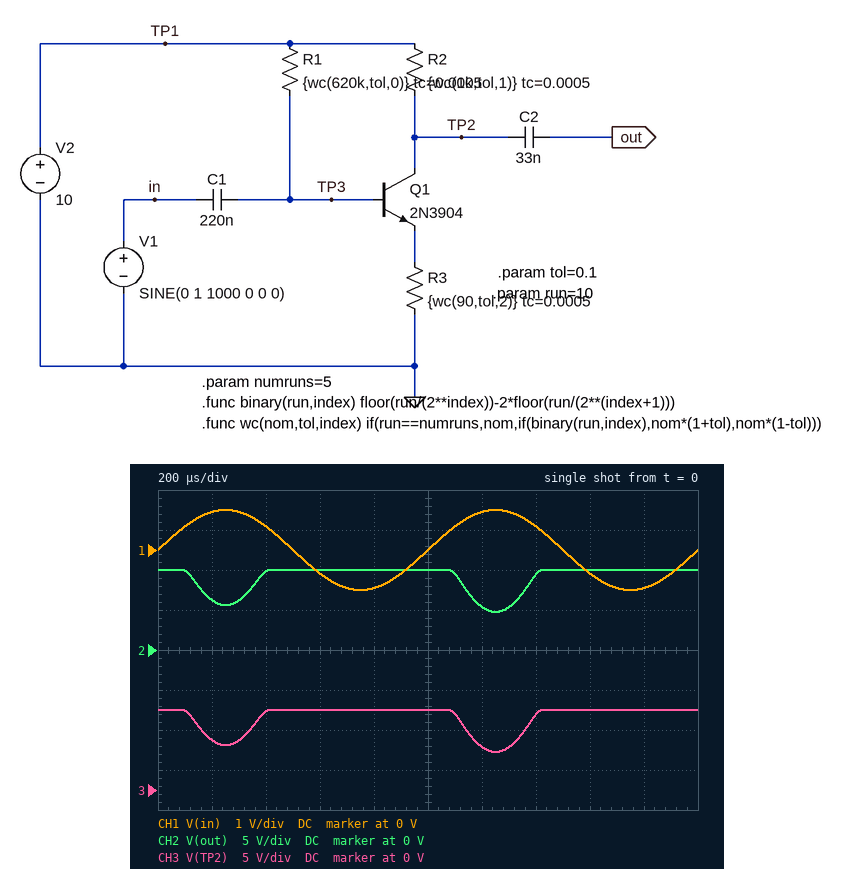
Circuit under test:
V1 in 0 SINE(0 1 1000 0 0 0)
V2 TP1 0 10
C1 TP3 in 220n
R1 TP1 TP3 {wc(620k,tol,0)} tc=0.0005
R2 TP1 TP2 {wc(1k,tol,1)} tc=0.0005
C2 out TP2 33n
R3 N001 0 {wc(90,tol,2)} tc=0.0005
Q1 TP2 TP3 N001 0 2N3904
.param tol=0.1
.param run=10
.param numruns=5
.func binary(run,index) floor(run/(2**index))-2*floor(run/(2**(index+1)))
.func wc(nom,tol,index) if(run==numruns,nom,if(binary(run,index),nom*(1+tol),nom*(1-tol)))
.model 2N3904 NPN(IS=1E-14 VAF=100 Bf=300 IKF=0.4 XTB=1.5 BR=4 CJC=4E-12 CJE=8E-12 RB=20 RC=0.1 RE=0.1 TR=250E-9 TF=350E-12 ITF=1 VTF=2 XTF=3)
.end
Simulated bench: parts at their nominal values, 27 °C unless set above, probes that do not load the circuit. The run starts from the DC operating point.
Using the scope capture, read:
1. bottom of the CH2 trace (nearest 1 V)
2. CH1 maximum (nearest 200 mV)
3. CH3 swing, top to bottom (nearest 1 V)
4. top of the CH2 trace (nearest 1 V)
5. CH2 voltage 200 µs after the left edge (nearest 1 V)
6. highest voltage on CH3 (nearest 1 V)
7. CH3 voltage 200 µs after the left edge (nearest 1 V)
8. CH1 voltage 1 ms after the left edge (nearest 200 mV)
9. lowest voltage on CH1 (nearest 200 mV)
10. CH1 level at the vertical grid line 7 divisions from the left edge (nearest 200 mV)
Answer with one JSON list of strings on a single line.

["5 V", "1.0 V", "5 V", "10 V", "6 V", "10 V", "6 V", "0 V", "-1.0 V", "600 mV"]
